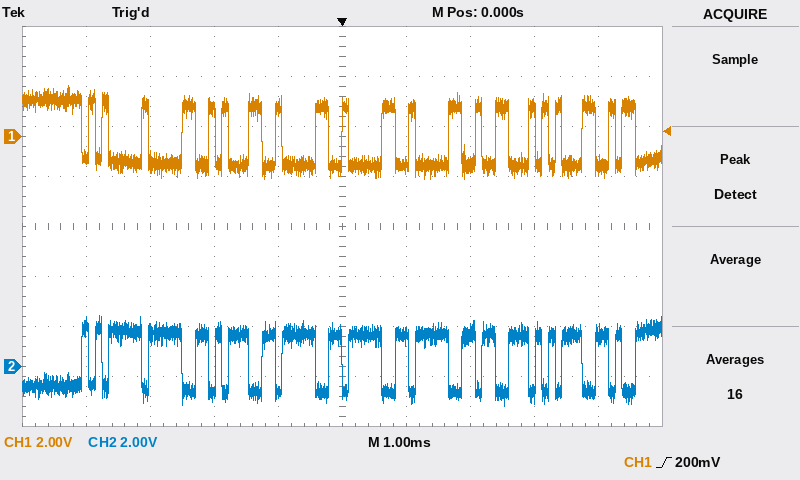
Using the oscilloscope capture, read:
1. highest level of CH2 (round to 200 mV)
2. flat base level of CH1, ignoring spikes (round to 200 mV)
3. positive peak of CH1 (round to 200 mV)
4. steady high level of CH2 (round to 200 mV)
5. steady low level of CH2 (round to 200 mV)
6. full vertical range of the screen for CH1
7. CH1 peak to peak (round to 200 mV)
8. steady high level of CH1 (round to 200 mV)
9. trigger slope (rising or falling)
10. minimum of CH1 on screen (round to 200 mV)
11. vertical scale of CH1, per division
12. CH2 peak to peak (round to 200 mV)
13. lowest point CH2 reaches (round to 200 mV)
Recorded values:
2.0 V
-1.2 V
2.0 V
1.2 V
-1.0 V
16 V
3.8 V
1.2 V
rising
-1.8 V
2 V
3.6 V
-1.6 V
